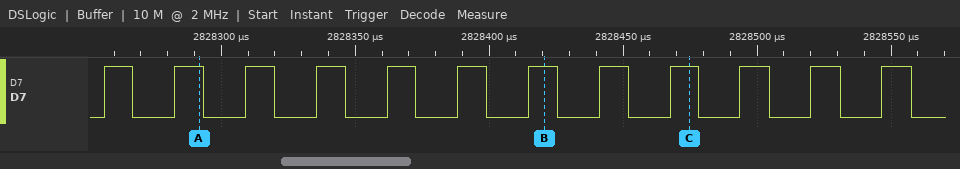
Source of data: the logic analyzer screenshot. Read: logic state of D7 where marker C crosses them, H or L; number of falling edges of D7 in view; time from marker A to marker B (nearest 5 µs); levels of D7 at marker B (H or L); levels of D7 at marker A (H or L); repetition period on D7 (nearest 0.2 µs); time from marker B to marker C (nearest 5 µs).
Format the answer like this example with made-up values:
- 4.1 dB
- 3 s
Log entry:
- D7=H
- 12
- 130 µs
- D7=H
- D7=H
- 26.4 µs
- 55 µs
